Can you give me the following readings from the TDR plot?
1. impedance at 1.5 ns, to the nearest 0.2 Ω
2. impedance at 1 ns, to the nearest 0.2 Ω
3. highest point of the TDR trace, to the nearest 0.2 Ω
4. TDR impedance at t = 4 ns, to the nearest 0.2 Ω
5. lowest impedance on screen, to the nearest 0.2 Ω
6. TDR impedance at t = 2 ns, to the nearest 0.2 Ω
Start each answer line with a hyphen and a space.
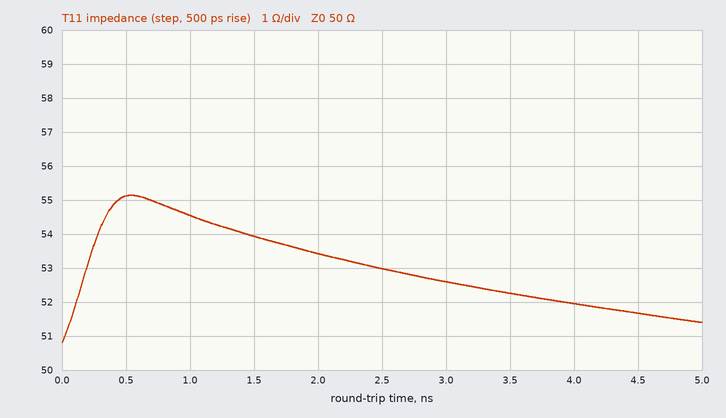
- 54.0 Ω
- 54.6 Ω
- 55.2 Ω
- 52.0 Ω
- 50.8 Ω
- 53.4 Ω
